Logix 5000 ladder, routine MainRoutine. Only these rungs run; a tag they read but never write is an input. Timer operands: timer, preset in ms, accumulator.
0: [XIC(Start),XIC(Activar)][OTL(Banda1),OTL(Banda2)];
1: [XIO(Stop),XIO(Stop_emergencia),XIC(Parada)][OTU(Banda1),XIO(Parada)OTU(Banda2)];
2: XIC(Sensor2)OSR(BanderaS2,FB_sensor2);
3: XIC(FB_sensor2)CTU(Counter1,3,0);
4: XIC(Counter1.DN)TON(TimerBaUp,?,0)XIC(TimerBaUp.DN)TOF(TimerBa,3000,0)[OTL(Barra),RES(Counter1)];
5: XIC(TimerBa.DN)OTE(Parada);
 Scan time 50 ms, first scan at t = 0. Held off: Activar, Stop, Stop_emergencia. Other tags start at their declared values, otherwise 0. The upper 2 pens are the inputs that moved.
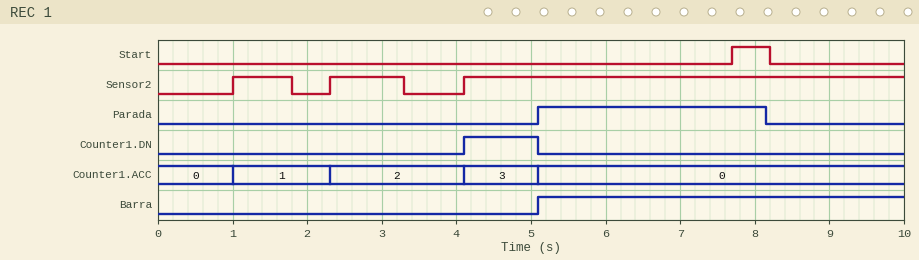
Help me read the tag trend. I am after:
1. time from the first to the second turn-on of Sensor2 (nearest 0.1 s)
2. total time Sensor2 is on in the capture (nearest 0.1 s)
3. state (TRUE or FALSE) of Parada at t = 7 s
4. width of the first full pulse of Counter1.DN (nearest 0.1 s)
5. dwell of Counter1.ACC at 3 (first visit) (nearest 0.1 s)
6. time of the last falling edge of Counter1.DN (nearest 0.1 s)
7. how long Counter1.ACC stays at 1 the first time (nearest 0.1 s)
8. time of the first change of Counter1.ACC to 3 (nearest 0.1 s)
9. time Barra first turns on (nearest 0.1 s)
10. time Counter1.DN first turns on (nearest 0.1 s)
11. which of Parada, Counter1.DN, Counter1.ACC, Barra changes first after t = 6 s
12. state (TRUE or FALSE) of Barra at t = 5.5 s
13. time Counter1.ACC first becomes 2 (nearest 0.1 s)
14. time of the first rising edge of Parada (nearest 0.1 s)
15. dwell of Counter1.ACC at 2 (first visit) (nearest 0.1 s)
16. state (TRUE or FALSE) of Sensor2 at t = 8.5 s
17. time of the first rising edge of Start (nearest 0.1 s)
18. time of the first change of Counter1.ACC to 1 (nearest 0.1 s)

1.3 s
7.7 s
TRUE
1.0 s
1.0 s
5.1 s
1.3 s
4.1 s
5.1 s
4.1 s
Parada
TRUE
2.3 s
5.1 s
1.8 s
TRUE
7.7 s
1.0 s
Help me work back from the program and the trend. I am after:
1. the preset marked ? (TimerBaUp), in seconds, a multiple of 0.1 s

1.0 s
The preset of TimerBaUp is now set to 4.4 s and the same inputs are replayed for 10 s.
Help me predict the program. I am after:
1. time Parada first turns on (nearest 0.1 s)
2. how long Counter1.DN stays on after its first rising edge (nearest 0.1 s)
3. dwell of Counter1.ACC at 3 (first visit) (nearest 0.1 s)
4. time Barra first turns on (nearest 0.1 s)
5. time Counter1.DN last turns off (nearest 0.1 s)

8.5 s
4.4 s
4.4 s
8.5 s
8.5 s
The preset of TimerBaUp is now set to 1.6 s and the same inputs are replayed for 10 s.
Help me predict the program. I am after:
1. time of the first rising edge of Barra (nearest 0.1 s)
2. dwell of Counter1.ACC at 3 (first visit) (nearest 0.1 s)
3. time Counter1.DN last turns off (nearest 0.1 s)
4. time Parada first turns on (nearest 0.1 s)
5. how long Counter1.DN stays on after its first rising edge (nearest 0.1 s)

5.7 s
1.6 s
5.7 s
5.7 s
1.6 s
